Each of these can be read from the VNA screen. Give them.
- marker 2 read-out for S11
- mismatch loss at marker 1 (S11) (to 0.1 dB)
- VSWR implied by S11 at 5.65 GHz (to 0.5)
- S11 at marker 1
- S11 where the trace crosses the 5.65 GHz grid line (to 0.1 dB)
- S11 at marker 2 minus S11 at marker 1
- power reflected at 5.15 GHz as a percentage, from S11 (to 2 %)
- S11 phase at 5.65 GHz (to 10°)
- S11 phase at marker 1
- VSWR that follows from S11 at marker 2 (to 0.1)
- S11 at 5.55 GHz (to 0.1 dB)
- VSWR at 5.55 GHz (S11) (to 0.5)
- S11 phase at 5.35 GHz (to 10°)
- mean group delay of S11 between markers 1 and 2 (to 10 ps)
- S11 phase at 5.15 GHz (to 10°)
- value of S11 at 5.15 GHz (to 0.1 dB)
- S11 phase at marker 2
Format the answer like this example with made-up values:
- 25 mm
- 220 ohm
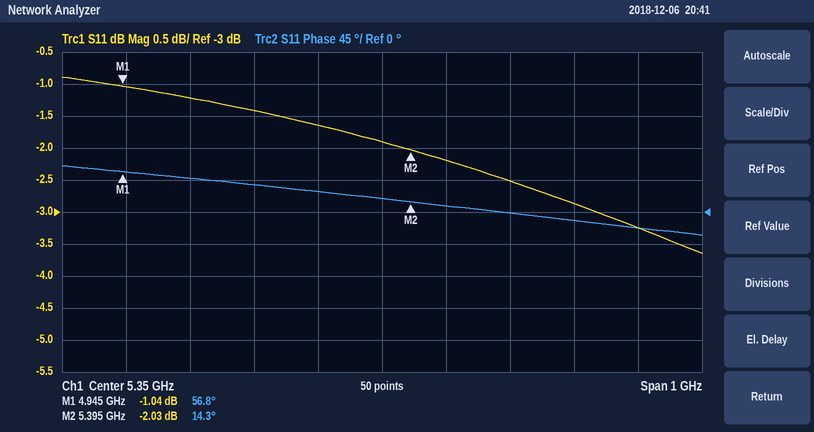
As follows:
- -2.03 dB
- 6.7 dB
- 6.0
- -1.04 dB
- -2.9 dB
- -0.99 dB
- 72 %
- -10°
- 56.8°
- 8.6
- -2.5 dB
- 7.0
- 20°
- 260 ps
- 40°
- -1.4 dB
- 14.3°
